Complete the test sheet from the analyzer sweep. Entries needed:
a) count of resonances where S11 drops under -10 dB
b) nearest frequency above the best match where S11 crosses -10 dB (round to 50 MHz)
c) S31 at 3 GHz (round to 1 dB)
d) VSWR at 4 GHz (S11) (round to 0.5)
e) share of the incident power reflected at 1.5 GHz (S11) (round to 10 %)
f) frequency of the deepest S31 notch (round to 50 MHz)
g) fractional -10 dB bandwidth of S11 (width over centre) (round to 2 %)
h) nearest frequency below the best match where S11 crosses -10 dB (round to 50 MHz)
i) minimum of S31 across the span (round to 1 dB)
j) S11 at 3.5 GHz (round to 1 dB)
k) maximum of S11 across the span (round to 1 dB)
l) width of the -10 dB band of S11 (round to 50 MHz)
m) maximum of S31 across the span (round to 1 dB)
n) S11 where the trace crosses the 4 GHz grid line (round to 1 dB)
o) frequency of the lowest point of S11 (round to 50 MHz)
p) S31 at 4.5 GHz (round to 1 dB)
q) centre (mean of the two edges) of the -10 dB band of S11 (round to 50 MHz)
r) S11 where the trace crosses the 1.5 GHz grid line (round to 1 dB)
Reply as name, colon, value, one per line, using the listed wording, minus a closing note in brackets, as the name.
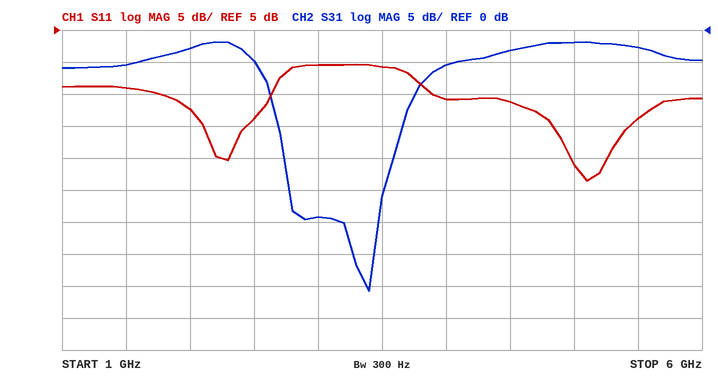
count of resonances where S11 drops under -10 dB: 2
nearest frequency above the best match where S11 crosses -10 dB: 5.45 GHz
S31 at 3 GHz: -29 dB
VSWR at 4 GHz (S11): 3.0
share of the incident power reflected at 1.5 GHz (S11): 40 %
frequency of the deepest S31 notch: 3.40 GHz
fractional -10 dB bandwidth of S11 (width over centre): 12 %
nearest frequency below the best match where S11 crosses -10 dB: 4.85 GHz
minimum of S31 across the span: -41 dB
S11 at 3.5 GHz: -1 dB
maximum of S11 across the span: 0 dB
width of the -10 dB band of S11: 600 MHz
maximum of S31 across the span: -2 dB
S11 where the trace crosses the 4 GHz grid line: -6 dB
frequency of the lowest point of S11: 5.10 GHz
S31 at 4.5 GHz: -3 dB
centre (mean of the two edges) of the -10 dB band of S11: 5.15 GHz
S11 where the trace crosses the 1.5 GHz grid line: -4 dB
